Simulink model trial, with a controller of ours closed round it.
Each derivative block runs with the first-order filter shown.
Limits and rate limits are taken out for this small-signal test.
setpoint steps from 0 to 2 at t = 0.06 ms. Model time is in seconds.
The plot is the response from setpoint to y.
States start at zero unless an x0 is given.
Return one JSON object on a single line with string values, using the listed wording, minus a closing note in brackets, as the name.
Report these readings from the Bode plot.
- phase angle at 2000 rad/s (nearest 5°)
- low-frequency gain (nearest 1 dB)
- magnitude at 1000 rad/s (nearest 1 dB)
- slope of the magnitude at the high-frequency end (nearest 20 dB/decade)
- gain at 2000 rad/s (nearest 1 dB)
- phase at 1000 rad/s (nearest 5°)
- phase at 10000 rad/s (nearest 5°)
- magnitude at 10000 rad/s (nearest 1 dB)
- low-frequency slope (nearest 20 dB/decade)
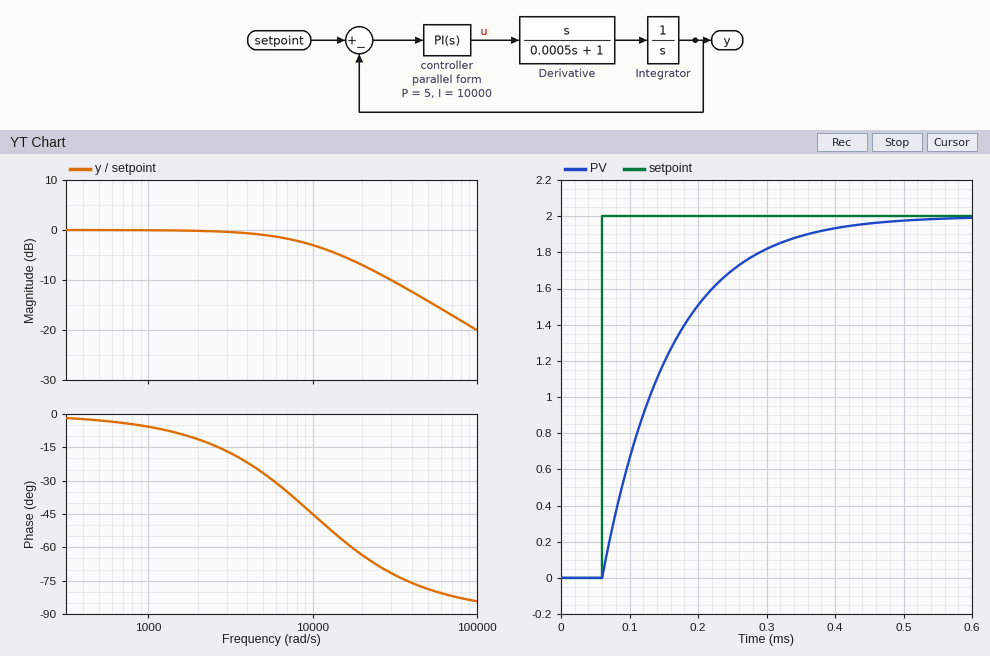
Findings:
{"phase angle at 2000 rad/s": "-10°", "low-frequency gain": "0 dB", "magnitude at 1000 rad/s": "0 dB", "slope of the magnitude at the high-frequency end": "-20 dB/decade", "gain at 2000 rad/s": "0 dB", "phase at 1000 rad/s": "-5°", "phase at 10000 rad/s": "-45°", "magnitude at 10000 rad/s": "-3 dB", "low-frequency slope": "0 dB/decade"}
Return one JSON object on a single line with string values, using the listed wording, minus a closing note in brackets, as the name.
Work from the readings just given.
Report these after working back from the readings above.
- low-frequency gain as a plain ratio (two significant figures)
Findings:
{"low-frequency gain as a plain ratio": "1.0"}
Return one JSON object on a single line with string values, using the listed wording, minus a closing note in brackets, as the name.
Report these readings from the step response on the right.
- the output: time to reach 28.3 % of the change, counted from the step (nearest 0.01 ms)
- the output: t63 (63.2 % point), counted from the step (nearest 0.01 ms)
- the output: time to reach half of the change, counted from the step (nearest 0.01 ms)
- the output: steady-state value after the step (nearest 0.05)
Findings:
{"the output: time to reach 28.3 % of the change, counted from the step": "0.03 ms", "the output: t63 (63.2 % point), counted from the step": "0.10 ms", "the output: time to reach half of the change, counted from the step": "0.07 ms", "the output: steady-state value after the step": "2.00"}
